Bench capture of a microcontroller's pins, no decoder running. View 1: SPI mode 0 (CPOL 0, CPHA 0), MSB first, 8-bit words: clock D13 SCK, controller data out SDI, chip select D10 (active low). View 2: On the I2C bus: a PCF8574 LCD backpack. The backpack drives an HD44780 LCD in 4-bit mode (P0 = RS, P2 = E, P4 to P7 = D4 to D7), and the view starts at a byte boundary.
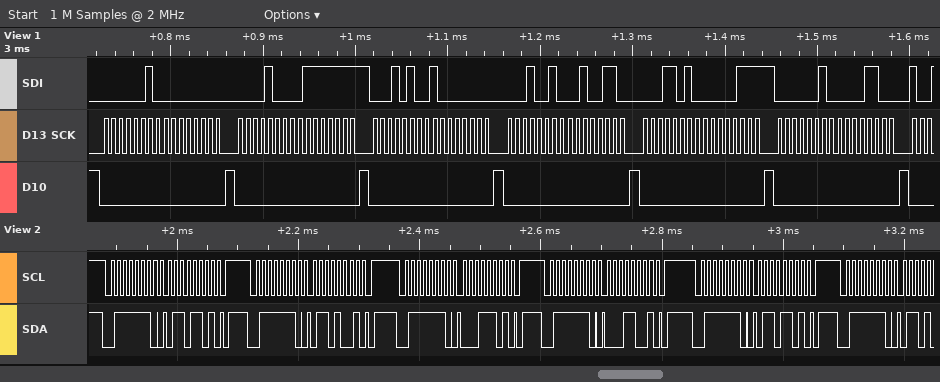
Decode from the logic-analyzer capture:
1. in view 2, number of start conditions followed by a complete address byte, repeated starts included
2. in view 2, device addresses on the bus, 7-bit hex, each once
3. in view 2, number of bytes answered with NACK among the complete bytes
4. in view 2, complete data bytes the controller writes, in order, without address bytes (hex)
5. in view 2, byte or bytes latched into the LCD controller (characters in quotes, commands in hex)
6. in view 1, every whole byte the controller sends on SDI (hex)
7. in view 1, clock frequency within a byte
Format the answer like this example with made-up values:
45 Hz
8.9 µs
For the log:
6
0x3F
0
6D 69 1D 19 6D
'a'
0x02 0x00 0x08 0x7F 0x14 0x80 0x12 0x26 0x1A 0x07 0x02 0x0C
125 kHz
